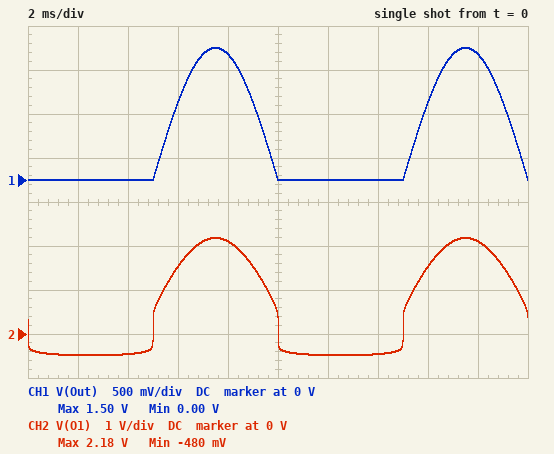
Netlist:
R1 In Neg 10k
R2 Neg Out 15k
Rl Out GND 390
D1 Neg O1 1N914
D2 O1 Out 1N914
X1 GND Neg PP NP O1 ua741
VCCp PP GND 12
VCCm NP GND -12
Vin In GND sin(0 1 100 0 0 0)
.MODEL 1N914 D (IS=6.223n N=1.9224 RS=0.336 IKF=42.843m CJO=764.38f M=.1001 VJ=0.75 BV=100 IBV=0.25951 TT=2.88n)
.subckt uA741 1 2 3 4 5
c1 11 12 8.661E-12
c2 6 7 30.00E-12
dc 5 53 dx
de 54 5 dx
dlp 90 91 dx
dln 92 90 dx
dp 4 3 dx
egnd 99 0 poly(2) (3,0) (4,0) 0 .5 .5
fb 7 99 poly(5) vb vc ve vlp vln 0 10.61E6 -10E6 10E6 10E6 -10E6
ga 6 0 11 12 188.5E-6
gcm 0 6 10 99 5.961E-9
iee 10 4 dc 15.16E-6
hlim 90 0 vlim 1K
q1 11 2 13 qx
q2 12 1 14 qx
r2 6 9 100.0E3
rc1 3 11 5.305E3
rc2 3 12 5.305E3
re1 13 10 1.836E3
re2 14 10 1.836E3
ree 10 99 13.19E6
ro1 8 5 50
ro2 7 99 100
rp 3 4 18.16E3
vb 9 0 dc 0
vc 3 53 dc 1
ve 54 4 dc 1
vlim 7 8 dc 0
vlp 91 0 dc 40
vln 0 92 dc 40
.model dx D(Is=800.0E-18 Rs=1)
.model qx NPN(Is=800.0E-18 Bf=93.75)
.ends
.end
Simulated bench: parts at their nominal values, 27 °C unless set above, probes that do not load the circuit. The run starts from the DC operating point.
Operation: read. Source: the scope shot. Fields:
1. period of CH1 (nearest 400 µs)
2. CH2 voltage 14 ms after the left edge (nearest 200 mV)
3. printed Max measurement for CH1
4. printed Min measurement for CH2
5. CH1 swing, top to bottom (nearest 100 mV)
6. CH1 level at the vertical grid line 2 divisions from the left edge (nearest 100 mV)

10.0 ms
-400 mV
1.50 V
-480 mV
1.5 V
0 V
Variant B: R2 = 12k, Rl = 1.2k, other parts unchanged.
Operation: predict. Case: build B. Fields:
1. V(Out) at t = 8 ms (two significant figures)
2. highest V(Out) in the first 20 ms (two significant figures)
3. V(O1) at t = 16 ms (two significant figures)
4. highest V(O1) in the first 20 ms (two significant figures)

1.1 V
1.2 V
1.3 V
1.8 V
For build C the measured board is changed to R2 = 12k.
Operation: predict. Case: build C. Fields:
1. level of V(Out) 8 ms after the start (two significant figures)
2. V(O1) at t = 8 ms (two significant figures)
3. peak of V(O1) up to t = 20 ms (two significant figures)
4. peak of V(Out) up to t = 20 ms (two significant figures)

1.1 V
1.8 V
1.9 V
1.2 V
